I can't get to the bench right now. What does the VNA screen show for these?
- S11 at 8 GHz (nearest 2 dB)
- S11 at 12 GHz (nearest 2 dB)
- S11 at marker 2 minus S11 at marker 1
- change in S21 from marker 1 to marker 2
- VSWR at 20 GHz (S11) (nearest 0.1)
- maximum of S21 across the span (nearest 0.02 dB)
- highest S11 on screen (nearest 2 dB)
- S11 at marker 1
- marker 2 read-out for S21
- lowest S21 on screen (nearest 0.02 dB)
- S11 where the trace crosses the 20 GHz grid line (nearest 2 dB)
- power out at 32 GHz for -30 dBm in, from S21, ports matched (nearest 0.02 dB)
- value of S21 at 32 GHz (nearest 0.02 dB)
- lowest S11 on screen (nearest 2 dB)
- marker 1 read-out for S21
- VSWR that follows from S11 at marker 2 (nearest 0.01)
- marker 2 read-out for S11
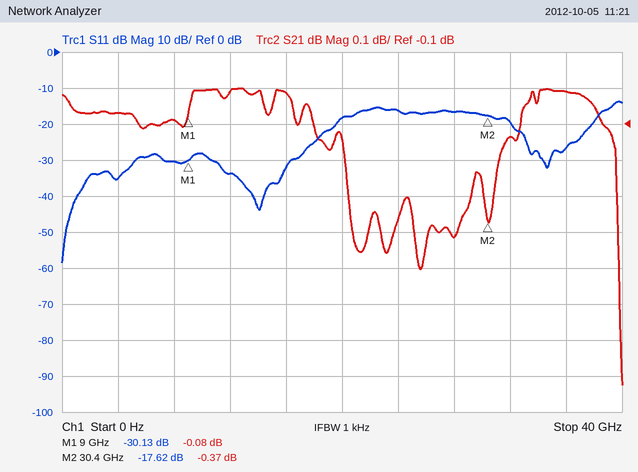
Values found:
-30 dB
-34 dB
12.51 dB
-0.29 dB
1.3
0.00 dB
-14 dB
-30.13 dB
-0.37 dB
-0.82 dB
-18 dB
-30.14 dBm
-0.14 dB
-58 dB
-0.08 dB
1.30
-17.62 dB
